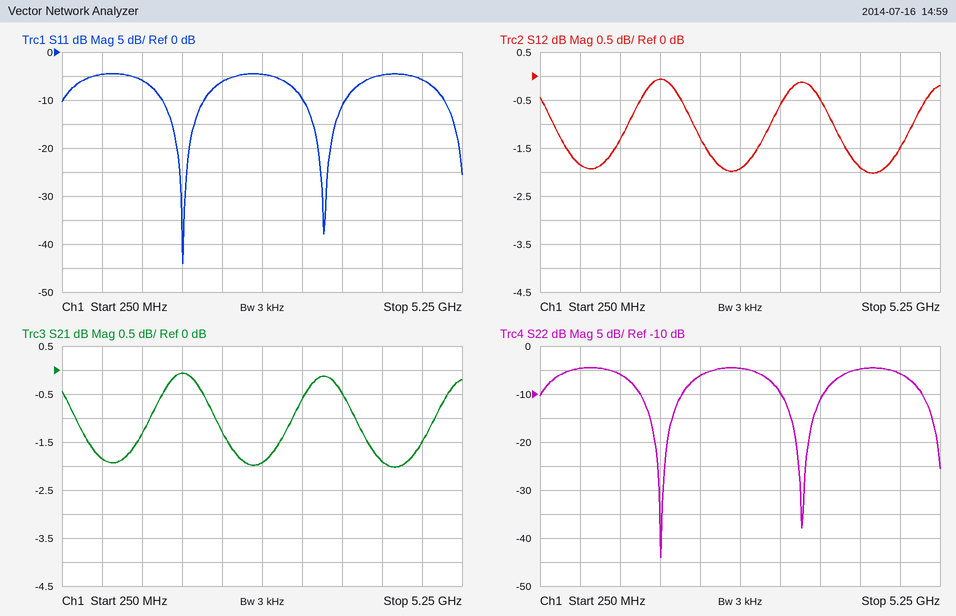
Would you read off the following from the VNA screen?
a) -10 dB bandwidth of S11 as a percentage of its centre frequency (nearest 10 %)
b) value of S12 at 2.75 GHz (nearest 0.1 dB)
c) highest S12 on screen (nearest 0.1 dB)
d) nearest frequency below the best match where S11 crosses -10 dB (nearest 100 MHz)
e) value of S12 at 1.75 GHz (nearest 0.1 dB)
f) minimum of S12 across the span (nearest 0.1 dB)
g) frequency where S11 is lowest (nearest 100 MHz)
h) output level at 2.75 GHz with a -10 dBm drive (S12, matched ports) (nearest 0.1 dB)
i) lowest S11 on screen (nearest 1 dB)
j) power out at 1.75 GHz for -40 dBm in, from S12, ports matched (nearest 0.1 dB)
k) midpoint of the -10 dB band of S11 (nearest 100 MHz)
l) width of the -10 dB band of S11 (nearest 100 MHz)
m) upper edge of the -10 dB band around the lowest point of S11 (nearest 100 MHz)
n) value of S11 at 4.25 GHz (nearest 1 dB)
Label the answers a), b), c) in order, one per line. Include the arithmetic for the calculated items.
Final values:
a) 500 MHz / 1.75 GHz ≈ 28.6 %, so 30 % to the nearest 10 %
b) -1.9 dB
c) -0.1 dB
d) 1.5 GHz
e) -0.1 dB
f) -2.0 dB
g) 1.8 GHz
h) -10 dBm + (-1.9 dB) = -11.9 dBm
i) -44 dB
j) -40 dBm + (-0.1 dB) = -40.1 dBm
k) 1.8 GHz
l) 2.0 GHz − 1.5 GHz = 500 MHz
m) 2.0 GHz
n) -5 dB
